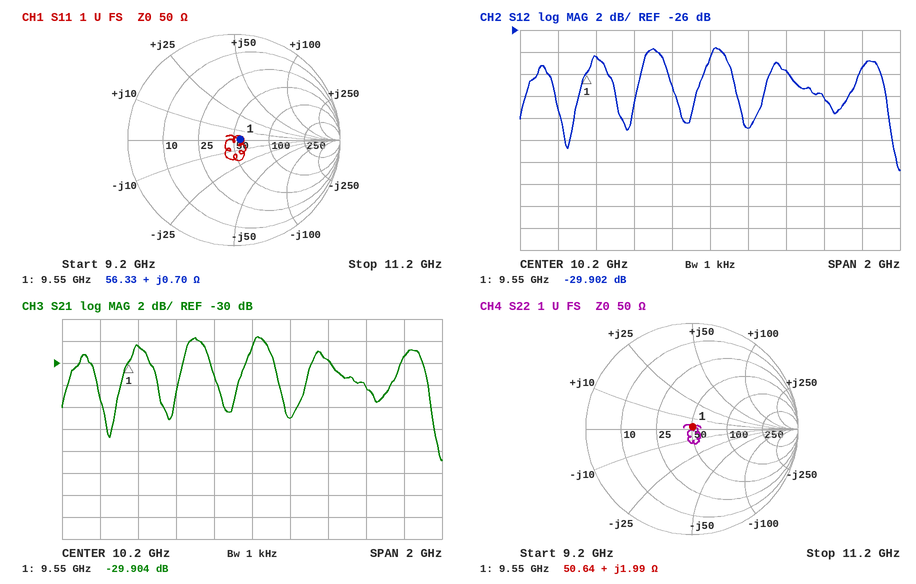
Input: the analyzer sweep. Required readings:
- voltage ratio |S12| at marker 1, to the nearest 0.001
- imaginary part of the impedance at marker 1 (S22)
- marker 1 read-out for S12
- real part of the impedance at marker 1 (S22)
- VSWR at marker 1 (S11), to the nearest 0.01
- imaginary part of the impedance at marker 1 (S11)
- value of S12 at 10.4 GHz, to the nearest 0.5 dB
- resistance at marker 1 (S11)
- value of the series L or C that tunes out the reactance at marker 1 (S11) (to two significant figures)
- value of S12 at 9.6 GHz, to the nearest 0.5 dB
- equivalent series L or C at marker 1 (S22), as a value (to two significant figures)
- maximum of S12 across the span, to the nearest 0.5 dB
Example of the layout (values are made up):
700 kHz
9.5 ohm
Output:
0.032
+1.99 Ω
-29.902 dB
50.64 Ω
1.13
+0.70 Ω
-35.0 dB
56.33 Ω
24 pF
-28.5 dB
33 pH
-27.5 dB
